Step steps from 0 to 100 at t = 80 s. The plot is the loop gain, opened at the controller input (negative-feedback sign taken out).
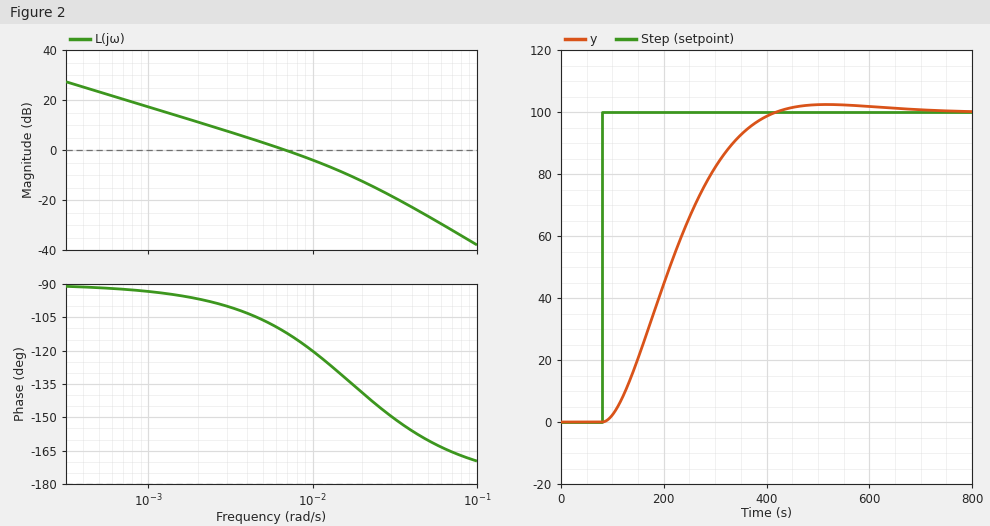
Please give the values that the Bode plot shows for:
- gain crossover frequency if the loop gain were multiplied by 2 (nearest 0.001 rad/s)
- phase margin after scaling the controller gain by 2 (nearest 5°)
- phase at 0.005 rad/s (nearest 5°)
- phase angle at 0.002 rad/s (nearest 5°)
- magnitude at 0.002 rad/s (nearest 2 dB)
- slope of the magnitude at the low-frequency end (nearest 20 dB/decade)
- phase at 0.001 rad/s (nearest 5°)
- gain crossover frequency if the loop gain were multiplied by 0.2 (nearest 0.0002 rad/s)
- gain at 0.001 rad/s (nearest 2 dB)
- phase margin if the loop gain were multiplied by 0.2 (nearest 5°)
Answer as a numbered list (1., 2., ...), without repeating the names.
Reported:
1. 0.012 rad/s
2. 55°
3. -105°
4. -95°
5. 12 dB
6. -20 dB/decade
7. -95°
8. 0.0014 rad/s
9. 18 dB
10. 85°
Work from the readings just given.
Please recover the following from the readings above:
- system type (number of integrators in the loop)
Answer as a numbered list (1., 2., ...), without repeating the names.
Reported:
1. 1
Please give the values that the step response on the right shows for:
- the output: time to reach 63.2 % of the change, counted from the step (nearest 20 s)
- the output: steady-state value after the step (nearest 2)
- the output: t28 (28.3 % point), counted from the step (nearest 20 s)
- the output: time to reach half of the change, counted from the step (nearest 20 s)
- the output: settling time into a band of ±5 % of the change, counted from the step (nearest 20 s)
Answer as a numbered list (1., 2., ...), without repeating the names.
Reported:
1. 160 s
2. 100
3. 80 s
4. 140 s
5. 280 s
